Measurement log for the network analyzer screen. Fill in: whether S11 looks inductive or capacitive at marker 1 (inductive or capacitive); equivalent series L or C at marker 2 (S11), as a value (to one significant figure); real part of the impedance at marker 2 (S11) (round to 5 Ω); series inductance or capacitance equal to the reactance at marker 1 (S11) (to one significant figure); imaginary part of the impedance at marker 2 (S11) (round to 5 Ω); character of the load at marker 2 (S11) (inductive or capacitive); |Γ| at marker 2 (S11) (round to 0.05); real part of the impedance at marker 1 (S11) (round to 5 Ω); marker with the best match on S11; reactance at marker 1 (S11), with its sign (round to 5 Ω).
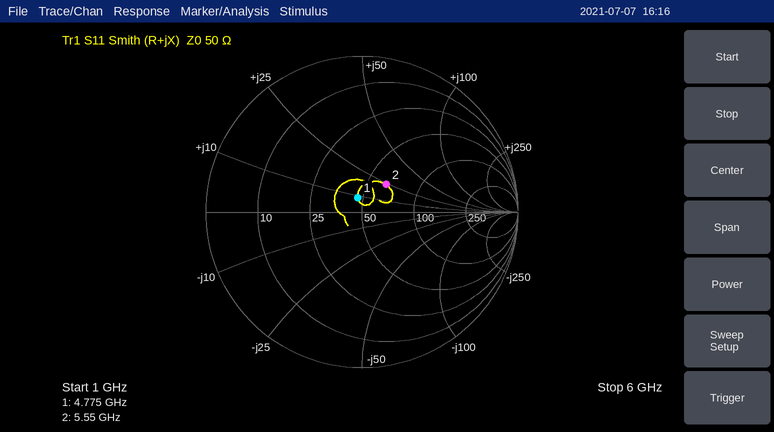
inductive
700 pH
65 Ω
300 pH
+25 Ω
inductive
0.25
45 Ω
marker 1
+10 Ω
